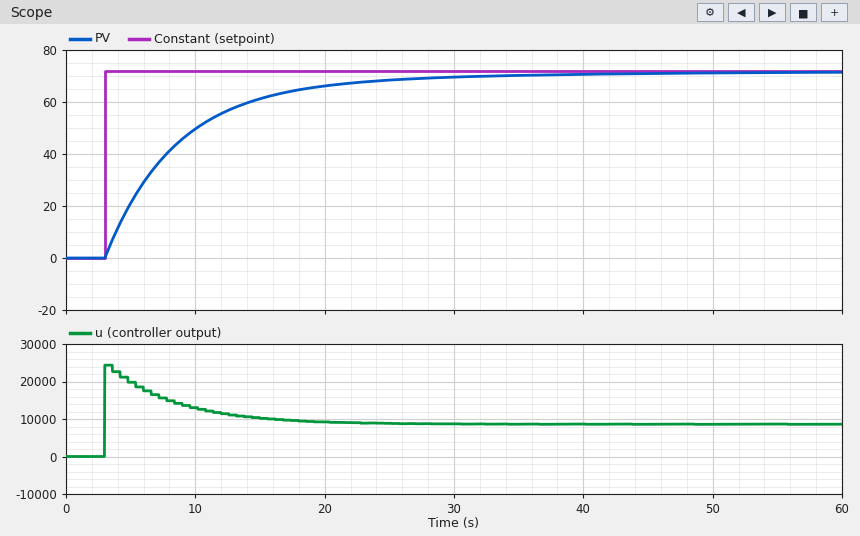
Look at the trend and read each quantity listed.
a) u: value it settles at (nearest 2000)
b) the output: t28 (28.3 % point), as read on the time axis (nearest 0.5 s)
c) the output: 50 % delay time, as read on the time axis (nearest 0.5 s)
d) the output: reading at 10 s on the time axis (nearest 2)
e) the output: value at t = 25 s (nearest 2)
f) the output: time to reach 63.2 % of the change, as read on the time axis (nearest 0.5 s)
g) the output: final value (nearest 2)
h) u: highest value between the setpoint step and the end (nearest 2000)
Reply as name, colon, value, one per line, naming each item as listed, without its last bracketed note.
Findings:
u: value it settles at: 8000
the output: t28 (28.3 % point), as read on the time axis: 5.0 s
the output: 50 % delay time, as read on the time axis: 7.0 s
the output: reading at 10 s on the time axis: 50
the output: value at t = 25 s: 68
the output: time to reach 63.2 % of the change, as read on the time axis: 9.0 s
the output: final value: 72
u: highest value between the setpoint step and the end: 24000
